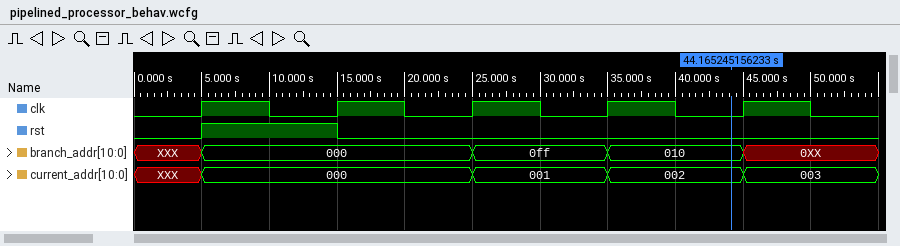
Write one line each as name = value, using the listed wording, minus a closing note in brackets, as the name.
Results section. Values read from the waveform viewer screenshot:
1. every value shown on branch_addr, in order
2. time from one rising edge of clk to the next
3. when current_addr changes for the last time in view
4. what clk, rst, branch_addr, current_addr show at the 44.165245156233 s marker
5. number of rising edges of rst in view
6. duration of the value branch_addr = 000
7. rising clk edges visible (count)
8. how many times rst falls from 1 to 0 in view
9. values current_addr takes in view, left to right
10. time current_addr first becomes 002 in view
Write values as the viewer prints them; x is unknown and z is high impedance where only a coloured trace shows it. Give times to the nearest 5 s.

every value shown on branch_addr, in order = XXX, 000, 0ff, 010, 0XX
time from one rising edge of clk to the next = 10 s
when current_addr changes for the last time in view = 45 s
what clk, rst, branch_addr, current_addr show at the 44.165245156233 s marker = clk=0, rst=0, branch_addr=010, current_addr=002
number of rising edges of rst in view = 1
duration of the value branch_addr = 000 = 20 s
rising clk edges visible = 5
how many times rst falls from 1 to 0 in view = 1
values current_addr takes in view, left to right = XXX, 000, 001, 002, 003
time current_addr first becomes 002 in view = 35 s
